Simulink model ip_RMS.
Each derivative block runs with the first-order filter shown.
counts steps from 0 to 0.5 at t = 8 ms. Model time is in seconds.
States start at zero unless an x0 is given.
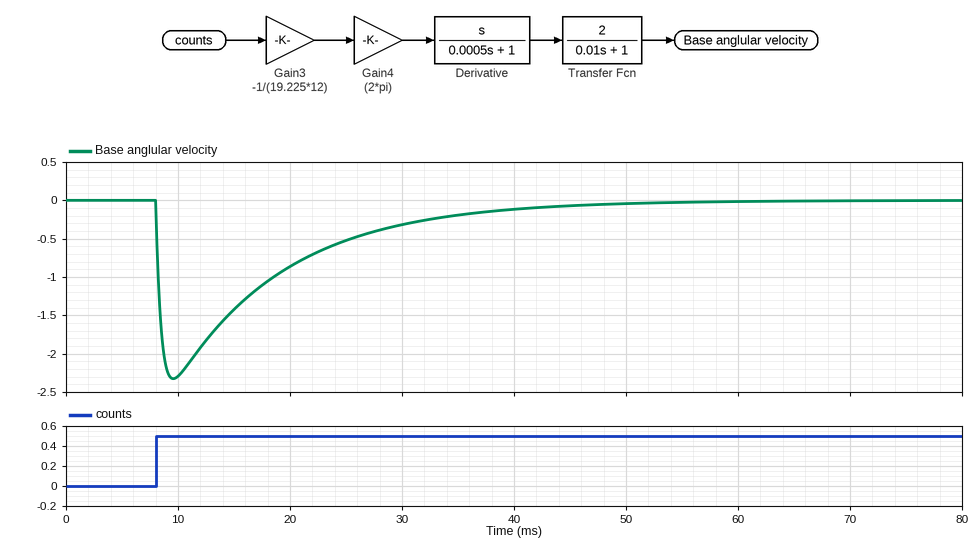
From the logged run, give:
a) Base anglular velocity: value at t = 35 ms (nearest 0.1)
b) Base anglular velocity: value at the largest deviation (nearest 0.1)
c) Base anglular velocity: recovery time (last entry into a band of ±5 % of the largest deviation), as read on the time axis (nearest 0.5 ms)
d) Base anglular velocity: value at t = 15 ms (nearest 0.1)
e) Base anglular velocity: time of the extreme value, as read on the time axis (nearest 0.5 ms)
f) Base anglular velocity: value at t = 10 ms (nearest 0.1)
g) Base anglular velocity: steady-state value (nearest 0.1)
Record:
-0.2
-2.3
40.0 ms
-1.4
9.5 ms
-2.3
0.0
